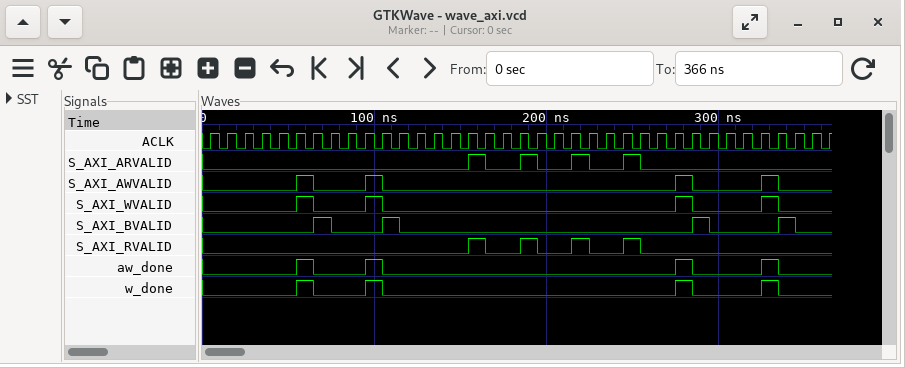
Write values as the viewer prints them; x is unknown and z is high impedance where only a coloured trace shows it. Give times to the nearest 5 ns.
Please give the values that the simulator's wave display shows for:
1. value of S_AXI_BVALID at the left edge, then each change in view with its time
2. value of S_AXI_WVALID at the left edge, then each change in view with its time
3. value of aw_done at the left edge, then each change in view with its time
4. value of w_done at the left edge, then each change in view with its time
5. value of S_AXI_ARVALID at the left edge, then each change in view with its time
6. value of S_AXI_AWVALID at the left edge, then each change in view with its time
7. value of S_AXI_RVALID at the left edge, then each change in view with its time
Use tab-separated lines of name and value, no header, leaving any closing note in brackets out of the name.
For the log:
value of S_AXI_BVALID at the left edge, then each change in view with its time	0, 1 at 65 ns, 0 at 75 ns, 1 at 105 ns, 0 at 115 ns, 1 at 285 ns, 0 at 295 ns, 1 at 335 ns, 0 at 345 ns
value of S_AXI_WVALID at the left edge, then each change in view with its time	0, 1 at 55 ns, 0 at 65 ns, 1 at 95 ns, 0 at 105 ns, 1 at 275 ns, 0 at 285 ns, 1 at 325 ns, 0 at 335 ns
value of aw_done at the left edge, then each change in view with its time	0, 1 at 55 ns, 0 at 65 ns, 1 at 95 ns, 0 at 105 ns, 1 at 275 ns, 0 at 285 ns, 1 at 325 ns, 0 at 335 ns
value of w_done at the left edge, then each change in view with its time	0, 1 at 55 ns, 0 at 65 ns, 1 at 95 ns, 0 at 105 ns, 1 at 275 ns, 0 at 285 ns, 1 at 325 ns, 0 at 335 ns
value of S_AXI_ARVALID at the left edge, then each change in view with its time	0, 1 at 155 ns, 0 at 165 ns, 1 at 185 ns, 0 at 195 ns, 1 at 215 ns, 0 at 225 ns, 1 at 245 ns, 0 at 255 ns
value of S_AXI_AWVALID at the left edge, then each change in view with its time	0, 1 at 55 ns, 0 at 65 ns, 1 at 95 ns, 0 at 105 ns, 1 at 275 ns, 0 at 285 ns, 1 at 325 ns, 0 at 335 ns
value of S_AXI_RVALID at the left edge, then each change in view with its time	0, 1 at 155 ns, 0 at 165 ns, 1 at 185 ns, 0 at 195 ns, 1 at 215 ns, 0 at 225 ns, 1 at 245 ns, 0 at 255 ns
